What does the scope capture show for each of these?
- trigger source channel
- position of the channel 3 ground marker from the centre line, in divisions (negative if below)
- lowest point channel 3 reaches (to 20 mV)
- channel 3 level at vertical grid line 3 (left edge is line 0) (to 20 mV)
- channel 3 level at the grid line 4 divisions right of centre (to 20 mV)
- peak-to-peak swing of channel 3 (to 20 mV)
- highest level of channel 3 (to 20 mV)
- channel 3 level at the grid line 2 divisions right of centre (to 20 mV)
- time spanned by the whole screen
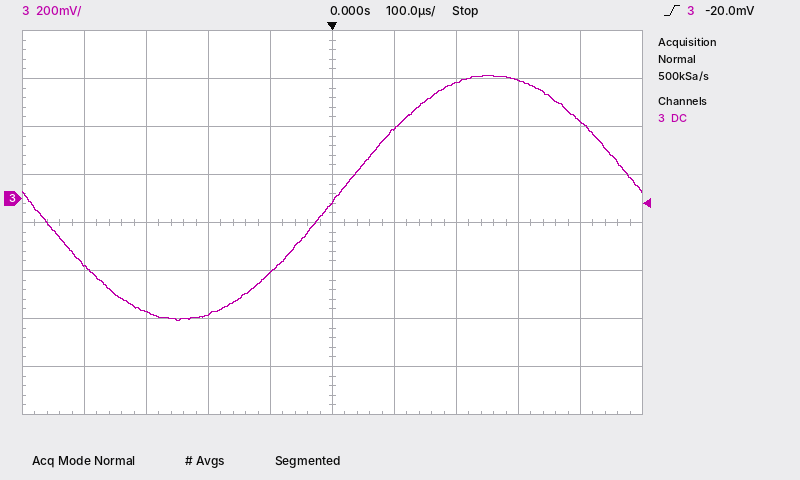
channel 3
+0.5 div
-500 mV
-480 mV
320 mV
1.02 V
520 mV
480 mV
1 ms
